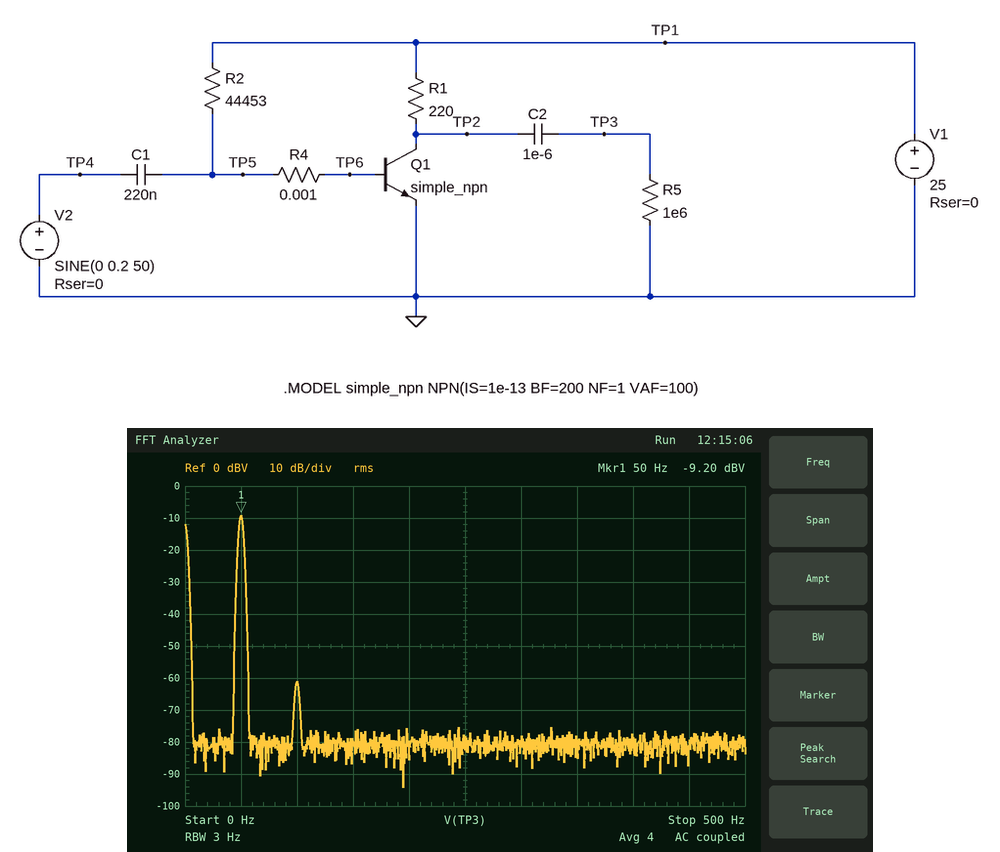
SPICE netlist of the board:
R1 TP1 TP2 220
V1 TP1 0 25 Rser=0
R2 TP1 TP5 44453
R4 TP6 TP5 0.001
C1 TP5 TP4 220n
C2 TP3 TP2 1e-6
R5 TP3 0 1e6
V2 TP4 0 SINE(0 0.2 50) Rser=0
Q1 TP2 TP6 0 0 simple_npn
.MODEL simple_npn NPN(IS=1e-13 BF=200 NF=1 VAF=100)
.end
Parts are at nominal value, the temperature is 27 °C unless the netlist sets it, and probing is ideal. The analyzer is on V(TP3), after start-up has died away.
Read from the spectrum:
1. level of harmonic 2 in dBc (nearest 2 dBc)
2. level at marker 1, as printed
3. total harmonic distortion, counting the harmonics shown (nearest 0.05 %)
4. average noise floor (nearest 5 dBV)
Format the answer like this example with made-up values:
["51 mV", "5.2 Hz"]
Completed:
["-52 dBc", "-9.20 dBV", "0.25 %", "-80 dBV"]
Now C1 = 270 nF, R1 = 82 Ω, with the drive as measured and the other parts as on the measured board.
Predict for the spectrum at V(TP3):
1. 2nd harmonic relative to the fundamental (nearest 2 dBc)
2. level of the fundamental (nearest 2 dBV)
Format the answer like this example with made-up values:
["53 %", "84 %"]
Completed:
["-58 dBc", "-14 dBV"]
